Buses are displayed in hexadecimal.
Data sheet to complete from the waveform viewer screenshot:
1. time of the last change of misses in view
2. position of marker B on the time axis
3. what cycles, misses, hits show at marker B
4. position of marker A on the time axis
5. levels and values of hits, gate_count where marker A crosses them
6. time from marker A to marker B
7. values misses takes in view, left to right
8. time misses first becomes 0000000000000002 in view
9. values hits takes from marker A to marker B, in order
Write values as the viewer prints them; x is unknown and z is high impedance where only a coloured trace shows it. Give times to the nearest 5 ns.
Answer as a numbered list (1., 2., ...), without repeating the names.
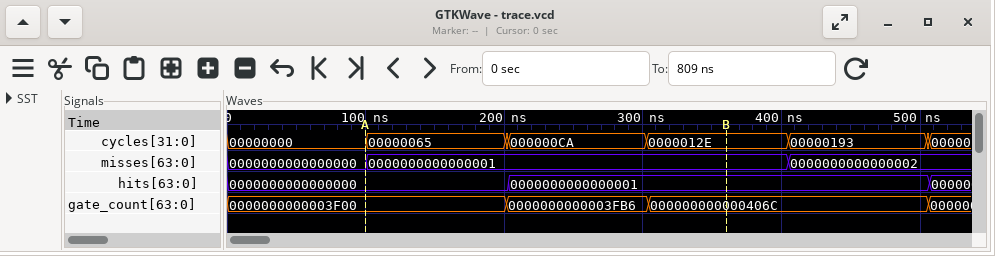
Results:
1. 405 ns
2. 360 ns
3. cycles=0000012E, misses=0000000000000001, hits=0000000000000001
4. 100 ns
5. hits=0000000000000000, gate_count=0000000000003F00
6. 260 ns
7. 0000000000000000, 0000000000000001, 0000000000000002
8. 405 ns
9. 0000000000000000, 0000000000000001
